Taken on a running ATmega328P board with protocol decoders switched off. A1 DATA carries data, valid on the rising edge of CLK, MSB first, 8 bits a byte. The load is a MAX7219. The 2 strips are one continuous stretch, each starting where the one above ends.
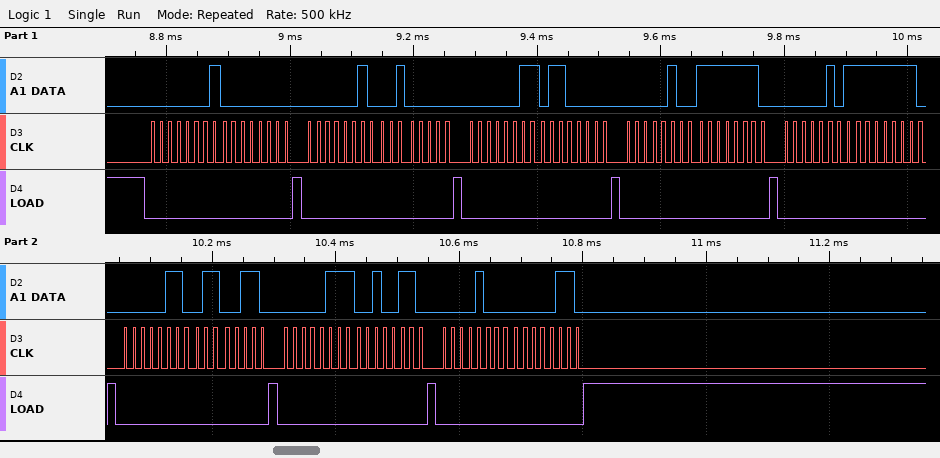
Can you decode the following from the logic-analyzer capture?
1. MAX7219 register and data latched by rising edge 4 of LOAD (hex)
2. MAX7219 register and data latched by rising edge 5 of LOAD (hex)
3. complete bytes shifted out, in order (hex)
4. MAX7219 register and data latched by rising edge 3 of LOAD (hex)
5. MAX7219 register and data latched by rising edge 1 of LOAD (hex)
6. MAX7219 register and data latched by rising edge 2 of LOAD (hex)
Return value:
register 0x4, data 0xFE
register 0x5, data 0xFE
0x01 0x00 0x02 0x20 0x03 0x60 0x04 0xFE 0x05 0xFE 0x06 0x66 0x07 0x26 0x08 0x06
register 0x3, data 0x60
register 0x1, data 0x00
register 0x2, data 0x20
